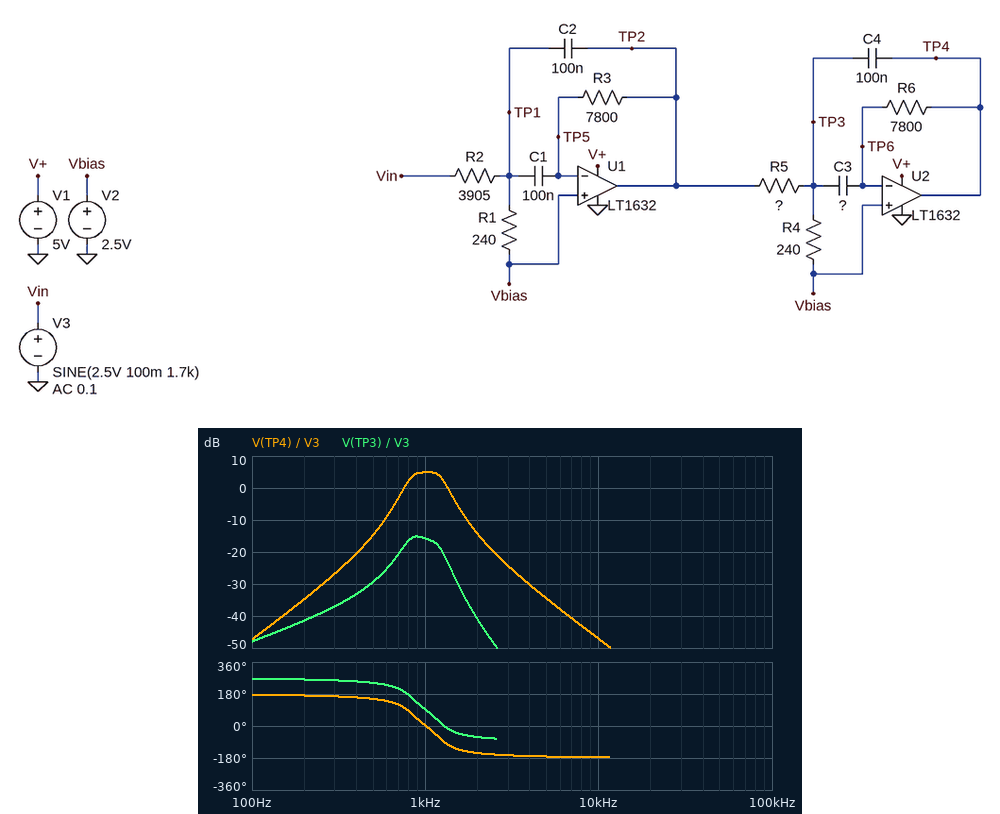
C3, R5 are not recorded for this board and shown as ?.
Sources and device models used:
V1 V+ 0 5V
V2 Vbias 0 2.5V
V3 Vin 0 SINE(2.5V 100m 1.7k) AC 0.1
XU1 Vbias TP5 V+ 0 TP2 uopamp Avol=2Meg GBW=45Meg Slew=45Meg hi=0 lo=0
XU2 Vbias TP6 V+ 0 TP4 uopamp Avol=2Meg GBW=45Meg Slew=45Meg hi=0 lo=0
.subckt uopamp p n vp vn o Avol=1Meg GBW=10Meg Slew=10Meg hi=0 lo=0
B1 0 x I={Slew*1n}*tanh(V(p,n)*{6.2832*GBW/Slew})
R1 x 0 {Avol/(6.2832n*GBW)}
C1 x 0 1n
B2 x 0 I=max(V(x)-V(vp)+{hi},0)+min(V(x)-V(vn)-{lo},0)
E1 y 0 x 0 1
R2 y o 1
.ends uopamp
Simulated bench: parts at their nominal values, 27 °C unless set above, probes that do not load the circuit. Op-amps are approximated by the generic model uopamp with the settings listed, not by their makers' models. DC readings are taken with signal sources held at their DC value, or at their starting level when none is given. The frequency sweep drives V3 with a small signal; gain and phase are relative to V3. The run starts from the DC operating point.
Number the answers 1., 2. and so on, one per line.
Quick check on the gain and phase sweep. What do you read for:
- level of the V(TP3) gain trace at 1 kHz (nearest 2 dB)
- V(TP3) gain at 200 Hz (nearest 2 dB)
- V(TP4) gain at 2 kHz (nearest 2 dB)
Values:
1. -16 dB
2. -42 dB
3. -14 dB
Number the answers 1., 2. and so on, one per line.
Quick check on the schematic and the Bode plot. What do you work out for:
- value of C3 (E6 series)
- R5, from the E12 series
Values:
1. 220 nF
2. 1.5 kΩ
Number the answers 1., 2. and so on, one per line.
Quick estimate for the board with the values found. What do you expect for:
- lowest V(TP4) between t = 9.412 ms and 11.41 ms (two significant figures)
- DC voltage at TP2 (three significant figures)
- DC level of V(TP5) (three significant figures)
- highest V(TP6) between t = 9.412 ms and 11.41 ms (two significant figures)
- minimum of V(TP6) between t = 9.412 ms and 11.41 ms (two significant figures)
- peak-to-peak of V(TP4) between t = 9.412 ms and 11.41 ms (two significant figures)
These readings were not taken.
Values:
1. 2.5 V
2. 2.50 V
3. 2.50 V
4. 2.5 V
5. 2.5 V
6. 69 mV
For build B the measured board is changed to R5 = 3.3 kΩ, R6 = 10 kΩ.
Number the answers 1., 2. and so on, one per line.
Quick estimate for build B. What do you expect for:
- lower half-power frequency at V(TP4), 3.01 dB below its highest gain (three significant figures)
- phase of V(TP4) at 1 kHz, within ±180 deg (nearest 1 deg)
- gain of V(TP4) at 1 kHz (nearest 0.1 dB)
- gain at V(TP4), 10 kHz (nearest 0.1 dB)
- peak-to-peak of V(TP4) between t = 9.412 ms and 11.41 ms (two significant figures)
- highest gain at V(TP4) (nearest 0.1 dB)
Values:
1. 657 Hz
2. -18 deg
3. -4.3 dB
4. -54.0 dB
5. 29 mV
6. -3.5 dB
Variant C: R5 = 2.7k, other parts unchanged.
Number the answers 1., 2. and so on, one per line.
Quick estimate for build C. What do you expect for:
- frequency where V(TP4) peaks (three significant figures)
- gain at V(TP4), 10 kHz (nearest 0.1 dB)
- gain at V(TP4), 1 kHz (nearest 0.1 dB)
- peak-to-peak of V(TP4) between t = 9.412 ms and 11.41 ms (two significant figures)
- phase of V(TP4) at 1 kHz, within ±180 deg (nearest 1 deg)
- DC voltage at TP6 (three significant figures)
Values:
1. 1.08 kHz
2. -52.2 dB
3. -0.9 dB
4. 38 mV
5. -1 deg
6. 2.50 V
